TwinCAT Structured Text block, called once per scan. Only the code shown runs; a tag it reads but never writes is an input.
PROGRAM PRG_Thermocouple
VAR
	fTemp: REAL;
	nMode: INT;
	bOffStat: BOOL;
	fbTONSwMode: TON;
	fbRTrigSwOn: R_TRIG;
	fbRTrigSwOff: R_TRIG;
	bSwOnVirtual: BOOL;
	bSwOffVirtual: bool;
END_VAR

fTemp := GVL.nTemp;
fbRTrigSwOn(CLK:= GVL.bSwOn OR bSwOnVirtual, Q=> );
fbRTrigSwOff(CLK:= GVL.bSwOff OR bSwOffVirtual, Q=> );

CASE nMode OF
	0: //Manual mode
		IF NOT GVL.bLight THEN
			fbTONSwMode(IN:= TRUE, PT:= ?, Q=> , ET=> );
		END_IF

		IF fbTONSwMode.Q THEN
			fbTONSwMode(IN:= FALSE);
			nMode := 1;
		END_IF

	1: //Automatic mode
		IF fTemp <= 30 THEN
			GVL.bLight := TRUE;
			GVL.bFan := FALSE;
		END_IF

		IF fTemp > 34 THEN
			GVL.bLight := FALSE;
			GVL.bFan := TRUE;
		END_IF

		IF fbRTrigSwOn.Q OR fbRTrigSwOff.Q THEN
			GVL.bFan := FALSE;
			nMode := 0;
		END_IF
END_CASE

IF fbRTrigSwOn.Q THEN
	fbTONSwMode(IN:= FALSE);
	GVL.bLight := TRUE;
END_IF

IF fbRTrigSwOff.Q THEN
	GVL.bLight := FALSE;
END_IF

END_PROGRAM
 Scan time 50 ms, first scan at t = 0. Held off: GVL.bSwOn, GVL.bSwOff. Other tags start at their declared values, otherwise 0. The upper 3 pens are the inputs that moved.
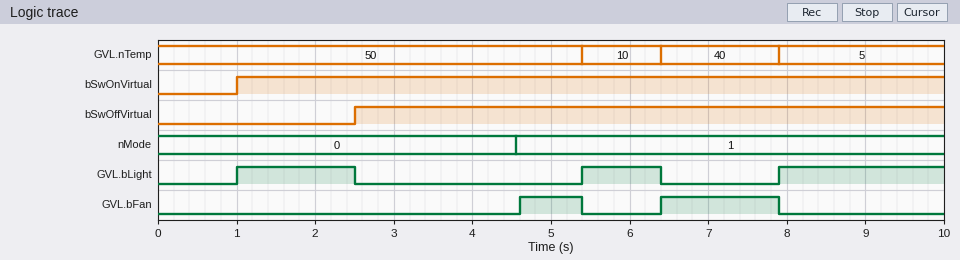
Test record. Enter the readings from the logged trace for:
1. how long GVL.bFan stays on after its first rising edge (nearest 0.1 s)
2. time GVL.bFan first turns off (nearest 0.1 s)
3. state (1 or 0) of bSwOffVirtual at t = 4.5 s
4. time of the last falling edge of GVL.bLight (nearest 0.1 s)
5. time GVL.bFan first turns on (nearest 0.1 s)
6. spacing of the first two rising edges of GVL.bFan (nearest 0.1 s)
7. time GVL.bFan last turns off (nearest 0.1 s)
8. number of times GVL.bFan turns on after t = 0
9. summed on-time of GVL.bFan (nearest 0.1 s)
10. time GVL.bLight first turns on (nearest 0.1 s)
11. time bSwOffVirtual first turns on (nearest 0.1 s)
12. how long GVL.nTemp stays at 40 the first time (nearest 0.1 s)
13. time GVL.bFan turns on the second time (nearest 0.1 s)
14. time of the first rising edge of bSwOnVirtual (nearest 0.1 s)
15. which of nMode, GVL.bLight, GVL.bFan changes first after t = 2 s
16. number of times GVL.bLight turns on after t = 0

0.8 s
5.4 s
1
6.4 s
4.6 s
1.8 s
7.9 s
2
2.3 s
1.0 s
2.5 s
1.5 s
6.4 s
1.0 s
GVL.bLight
3
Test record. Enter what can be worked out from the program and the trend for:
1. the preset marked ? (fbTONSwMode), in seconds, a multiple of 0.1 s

2.0 s
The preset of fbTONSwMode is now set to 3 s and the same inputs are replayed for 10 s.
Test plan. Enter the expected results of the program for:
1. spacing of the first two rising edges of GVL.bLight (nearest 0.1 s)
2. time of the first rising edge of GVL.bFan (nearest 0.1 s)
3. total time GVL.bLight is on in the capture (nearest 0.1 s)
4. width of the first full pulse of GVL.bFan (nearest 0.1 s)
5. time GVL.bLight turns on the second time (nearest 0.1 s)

4.6 s
6.4 s
4.4 s
1.5 s
5.6 s
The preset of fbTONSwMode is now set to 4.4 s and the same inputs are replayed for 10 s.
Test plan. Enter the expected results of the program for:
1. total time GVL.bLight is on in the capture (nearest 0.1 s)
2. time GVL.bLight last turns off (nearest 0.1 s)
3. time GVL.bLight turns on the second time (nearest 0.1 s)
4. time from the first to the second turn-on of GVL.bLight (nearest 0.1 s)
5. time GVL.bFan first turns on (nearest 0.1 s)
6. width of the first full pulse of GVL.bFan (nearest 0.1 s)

3.6 s
2.5 s
7.9 s
6.9 s
7.0 s
0.9 s
